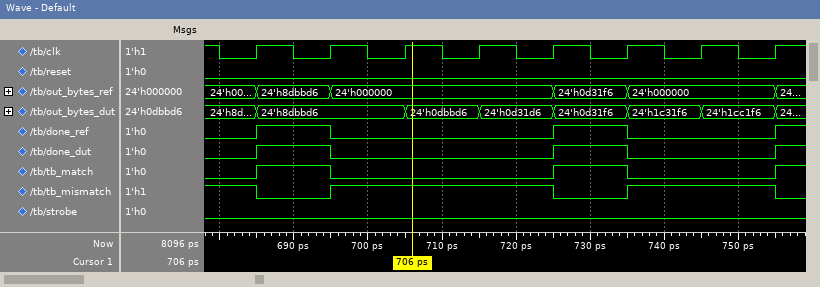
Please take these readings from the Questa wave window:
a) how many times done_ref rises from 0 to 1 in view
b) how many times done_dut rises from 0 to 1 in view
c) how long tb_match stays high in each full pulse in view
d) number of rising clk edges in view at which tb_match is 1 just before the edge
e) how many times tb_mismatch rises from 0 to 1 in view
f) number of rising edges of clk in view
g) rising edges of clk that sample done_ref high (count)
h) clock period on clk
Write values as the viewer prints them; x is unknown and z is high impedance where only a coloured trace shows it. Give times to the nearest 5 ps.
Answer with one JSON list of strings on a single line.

["3", "3", "10 ps, 10 ps", "2", "2", "8", "2", "10 ps"]
